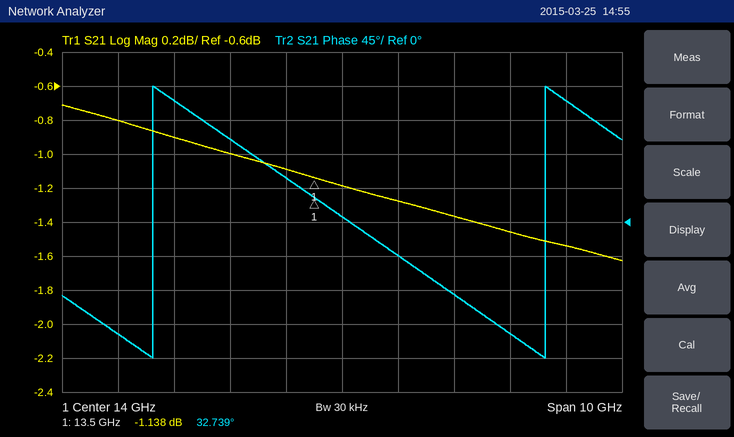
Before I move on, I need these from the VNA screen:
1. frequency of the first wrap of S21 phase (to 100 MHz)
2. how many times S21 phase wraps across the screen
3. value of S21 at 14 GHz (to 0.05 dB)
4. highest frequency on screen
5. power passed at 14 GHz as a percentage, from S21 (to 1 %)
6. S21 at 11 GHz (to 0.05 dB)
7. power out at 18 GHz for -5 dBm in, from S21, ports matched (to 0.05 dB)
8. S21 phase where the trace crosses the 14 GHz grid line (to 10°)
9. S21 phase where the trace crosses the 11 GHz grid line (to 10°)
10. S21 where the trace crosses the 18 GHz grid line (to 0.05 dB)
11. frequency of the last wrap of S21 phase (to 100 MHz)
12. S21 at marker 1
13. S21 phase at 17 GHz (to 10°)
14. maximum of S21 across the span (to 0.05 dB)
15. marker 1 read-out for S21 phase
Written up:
10.6 GHz
2
-1.20 dB
19 GHz
76 %
-0.90 dB
-6.55 dBm
10°
160°
-1.55 dB
17.6 GHz
-1.138 dB
-150°
-0.70 dB
32.739°
